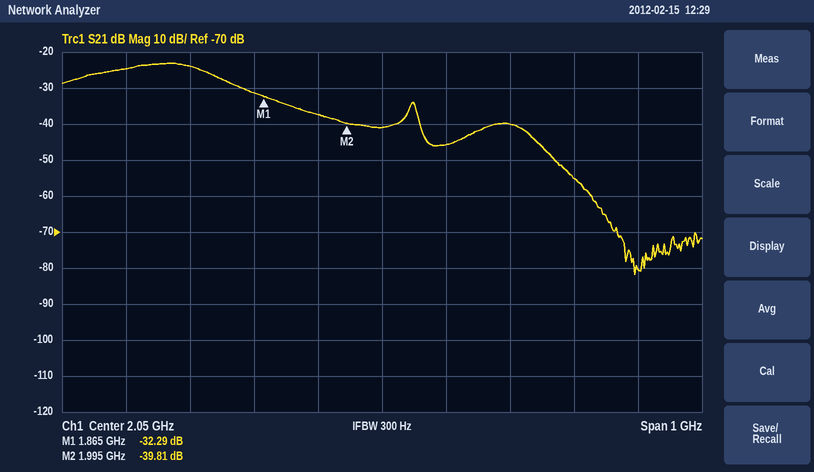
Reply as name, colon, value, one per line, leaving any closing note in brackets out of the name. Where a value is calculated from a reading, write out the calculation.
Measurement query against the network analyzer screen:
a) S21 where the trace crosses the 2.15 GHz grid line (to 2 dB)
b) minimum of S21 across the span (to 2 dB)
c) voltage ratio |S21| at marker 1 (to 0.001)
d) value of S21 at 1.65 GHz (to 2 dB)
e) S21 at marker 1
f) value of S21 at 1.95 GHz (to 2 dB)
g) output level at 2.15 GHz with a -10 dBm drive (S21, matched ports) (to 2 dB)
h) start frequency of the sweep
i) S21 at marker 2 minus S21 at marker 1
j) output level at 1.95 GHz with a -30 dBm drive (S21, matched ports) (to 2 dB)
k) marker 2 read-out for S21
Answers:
S21 where the trace crosses the 2.15 GHz grid line: -46 dB
minimum of S21 across the span: -82 dB
voltage ratio |S21| at marker 1: 10^(-32.29/20) ≈ 0.024
value of S21 at 1.65 GHz: -24 dB
S21 at marker 1: -32.29 dB
value of S21 at 1.95 GHz: -38 dB
output level at 2.15 GHz with a -10 dBm drive (S21, matched ports): -10 dBm + (-46 dB) = -56 dBm
start frequency of the sweep: 1.55 GHz
S21 at marker 2 minus S21 at marker 1: -39.81 − (-32.29) = -7.52 dB
output level at 1.95 GHz with a -30 dBm drive (S21, matched ports): -30 dBm + (-38 dB) = -68 dBm
marker 2 read-out for S21: -39.81 dB
